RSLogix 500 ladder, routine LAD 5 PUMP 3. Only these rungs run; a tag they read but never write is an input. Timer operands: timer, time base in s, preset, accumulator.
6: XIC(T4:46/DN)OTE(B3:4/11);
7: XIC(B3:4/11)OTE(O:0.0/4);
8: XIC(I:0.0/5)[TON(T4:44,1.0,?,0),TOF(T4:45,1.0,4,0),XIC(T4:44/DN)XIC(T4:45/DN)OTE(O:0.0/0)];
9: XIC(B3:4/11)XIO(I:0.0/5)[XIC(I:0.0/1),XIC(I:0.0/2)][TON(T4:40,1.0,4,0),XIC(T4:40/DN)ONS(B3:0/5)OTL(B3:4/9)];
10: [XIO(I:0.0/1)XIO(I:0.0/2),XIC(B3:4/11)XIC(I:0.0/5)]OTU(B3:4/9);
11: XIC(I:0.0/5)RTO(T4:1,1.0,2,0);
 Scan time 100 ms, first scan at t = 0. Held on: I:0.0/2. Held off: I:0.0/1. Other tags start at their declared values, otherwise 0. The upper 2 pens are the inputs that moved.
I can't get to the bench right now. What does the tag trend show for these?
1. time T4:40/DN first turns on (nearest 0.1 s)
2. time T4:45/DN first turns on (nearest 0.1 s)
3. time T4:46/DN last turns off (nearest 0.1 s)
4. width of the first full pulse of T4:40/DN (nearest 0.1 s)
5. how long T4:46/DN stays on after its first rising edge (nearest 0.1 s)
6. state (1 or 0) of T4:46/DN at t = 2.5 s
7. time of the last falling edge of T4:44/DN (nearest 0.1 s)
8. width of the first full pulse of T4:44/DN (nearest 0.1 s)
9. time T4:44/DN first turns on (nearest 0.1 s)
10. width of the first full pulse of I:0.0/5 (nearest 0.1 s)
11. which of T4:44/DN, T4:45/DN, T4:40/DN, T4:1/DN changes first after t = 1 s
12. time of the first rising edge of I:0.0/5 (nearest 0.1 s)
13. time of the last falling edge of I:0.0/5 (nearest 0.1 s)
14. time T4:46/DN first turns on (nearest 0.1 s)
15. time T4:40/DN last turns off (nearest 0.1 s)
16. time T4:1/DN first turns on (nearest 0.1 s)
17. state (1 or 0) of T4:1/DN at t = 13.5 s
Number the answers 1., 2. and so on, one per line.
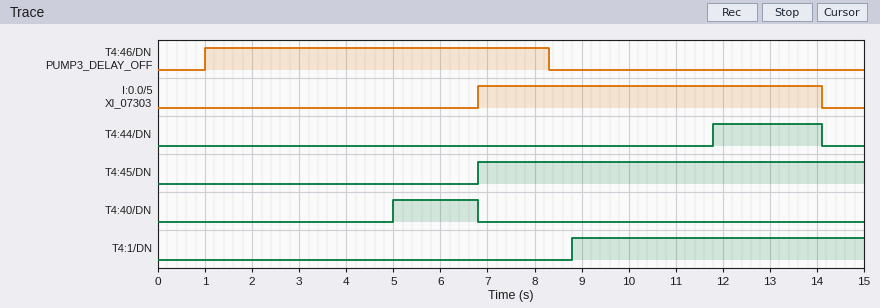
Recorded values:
1. 5.0 s
2. 6.8 s
3. 8.3 s
4. 1.8 s
5. 7.3 s
6. 1
7. 14.1 s
8. 2.3 s
9. 11.8 s
10. 7.3 s
11. T4:40/DN
12. 6.8 s
13. 14.1 s
14. 1.0 s
15. 6.8 s
16. 8.8 s
17. 1
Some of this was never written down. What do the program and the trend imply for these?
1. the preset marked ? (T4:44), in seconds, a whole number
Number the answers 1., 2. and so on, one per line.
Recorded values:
1. 5 s
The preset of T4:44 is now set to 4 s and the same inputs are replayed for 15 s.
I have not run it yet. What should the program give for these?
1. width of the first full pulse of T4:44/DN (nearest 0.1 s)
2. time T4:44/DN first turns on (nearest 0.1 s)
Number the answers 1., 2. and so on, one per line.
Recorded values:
1. 3.3 s
2. 10.8 s
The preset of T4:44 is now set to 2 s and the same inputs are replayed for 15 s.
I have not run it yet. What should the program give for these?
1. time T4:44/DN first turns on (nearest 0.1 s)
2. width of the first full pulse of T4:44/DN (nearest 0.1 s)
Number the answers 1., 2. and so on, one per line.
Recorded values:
1. 8.8 s
2. 5.3 s
